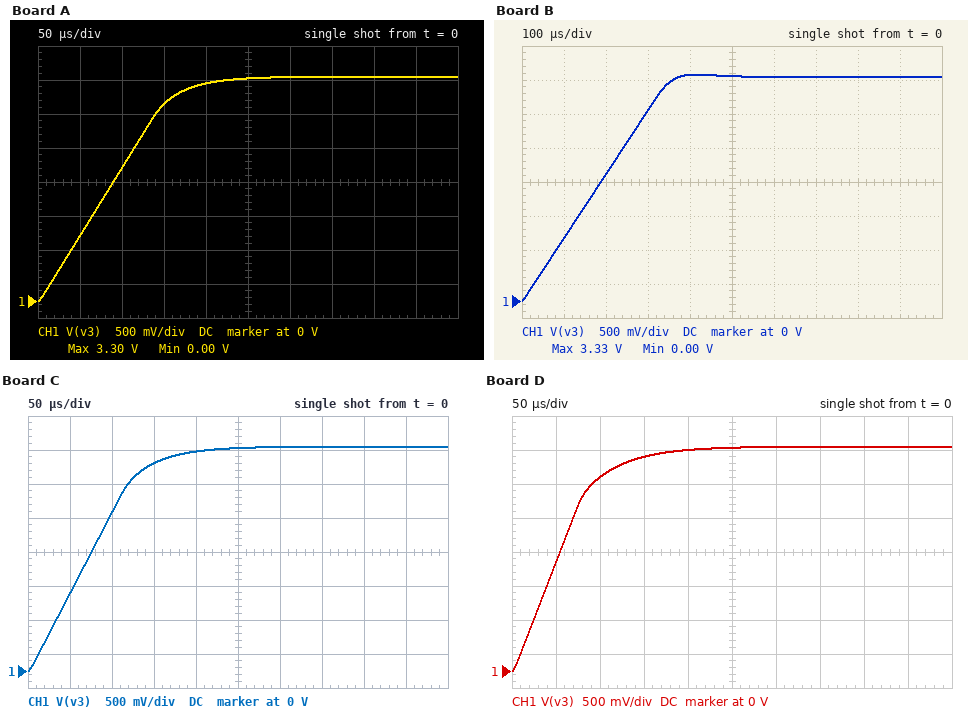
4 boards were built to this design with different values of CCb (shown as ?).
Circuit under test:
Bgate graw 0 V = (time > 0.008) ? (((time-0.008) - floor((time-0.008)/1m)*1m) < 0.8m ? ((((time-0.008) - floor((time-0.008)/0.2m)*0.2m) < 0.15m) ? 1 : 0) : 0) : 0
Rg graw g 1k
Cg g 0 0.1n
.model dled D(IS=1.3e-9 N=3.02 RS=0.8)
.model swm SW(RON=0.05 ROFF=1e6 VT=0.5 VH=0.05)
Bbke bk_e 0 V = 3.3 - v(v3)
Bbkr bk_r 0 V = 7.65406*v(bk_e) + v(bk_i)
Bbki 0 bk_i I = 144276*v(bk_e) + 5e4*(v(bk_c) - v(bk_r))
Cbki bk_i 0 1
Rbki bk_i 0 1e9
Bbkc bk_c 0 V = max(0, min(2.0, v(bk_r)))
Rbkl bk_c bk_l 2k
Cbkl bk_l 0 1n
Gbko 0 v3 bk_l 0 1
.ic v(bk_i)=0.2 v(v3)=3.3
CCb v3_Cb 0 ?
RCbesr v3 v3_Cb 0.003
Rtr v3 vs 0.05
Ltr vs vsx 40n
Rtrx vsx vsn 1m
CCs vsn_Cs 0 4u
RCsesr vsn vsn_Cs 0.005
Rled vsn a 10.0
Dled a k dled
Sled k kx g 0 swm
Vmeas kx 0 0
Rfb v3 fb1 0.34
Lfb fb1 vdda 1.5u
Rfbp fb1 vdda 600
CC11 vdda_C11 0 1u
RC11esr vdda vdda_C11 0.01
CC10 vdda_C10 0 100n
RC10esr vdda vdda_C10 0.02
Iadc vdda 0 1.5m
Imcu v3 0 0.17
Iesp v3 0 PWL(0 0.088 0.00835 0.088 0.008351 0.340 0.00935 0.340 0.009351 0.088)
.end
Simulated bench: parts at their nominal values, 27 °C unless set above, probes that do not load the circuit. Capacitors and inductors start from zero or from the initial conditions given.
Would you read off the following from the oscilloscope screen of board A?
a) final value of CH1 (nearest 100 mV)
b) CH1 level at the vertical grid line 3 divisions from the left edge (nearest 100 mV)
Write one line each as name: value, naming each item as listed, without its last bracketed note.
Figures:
final value of CH1: 3.3 V
CH1 level at the vertical grid line 3 divisions from the left edge: 2.9 V
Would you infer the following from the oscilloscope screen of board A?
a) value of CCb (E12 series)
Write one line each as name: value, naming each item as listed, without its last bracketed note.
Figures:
value of CCb: 82 µF
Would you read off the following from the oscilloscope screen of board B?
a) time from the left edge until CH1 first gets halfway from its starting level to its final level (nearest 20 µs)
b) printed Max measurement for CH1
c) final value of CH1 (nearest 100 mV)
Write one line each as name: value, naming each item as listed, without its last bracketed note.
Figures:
time from the left edge until CH1 first gets halfway from its starting level to its final level: 180 µs
printed Max measurement for CH1: 3.33 V
final value of CH1: 3.3 V
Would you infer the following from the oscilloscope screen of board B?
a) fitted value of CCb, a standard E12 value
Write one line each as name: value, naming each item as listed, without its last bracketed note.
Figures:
fitted value of CCb, a standard E12 value: 180 µF
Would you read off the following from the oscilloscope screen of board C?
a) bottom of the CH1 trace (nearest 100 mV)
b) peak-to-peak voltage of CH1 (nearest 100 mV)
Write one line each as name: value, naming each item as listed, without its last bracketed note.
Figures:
bottom of the CH1 trace: 0 V
peak-to-peak voltage of CH1: 3.3 V
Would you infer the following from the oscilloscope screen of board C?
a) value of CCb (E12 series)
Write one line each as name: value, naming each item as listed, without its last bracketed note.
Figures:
value of CCb: 68 µF
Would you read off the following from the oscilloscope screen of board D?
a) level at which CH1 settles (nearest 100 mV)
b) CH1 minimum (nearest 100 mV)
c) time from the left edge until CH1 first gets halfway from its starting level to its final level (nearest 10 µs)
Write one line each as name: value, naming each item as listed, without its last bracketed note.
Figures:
level at which CH1 settles: 3.3 V
CH1 minimum: 0 V
time from the left edge until CH1 first gets halfway from its starting level to its final level: 50 µs
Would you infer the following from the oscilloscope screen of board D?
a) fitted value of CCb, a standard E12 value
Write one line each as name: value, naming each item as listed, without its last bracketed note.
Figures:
fitted value of CCb, a standard E12 value: 47 µF
